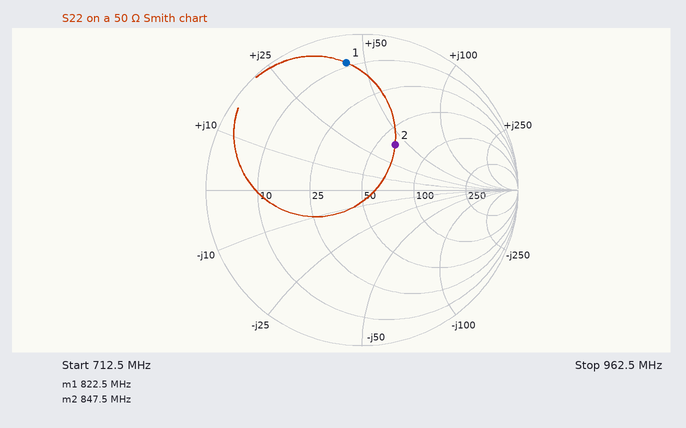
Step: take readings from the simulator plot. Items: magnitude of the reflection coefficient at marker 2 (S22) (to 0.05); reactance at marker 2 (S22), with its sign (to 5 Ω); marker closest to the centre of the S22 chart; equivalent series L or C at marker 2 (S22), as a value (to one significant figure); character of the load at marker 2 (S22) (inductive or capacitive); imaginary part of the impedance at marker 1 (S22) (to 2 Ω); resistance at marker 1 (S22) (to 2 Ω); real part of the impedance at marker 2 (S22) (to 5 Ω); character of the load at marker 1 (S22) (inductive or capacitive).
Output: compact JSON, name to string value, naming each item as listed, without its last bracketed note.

{"magnitude of the reflection coefficient at marker 2 (S22)": "0.35", "reactance at marker 2 (S22), with its sign": "+40 Ω", "marker closest to the centre of the S22 chart": "marker 2", "equivalent series L or C at marker 2 (S22), as a value": "8 nH", "character of the load at marker 2 (S22)": "inductive", "imaginary part of the impedance at marker 1 (S22)": "+44 Ω", "resistance at marker 1 (S22)": "8 Ω", "real part of the impedance at marker 2 (S22)": "60 Ω", "character of the load at marker 1 (S22)": "inductive"}
